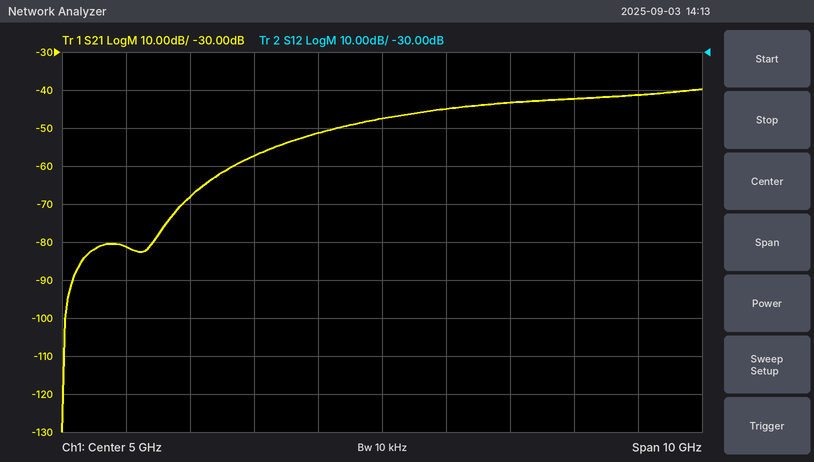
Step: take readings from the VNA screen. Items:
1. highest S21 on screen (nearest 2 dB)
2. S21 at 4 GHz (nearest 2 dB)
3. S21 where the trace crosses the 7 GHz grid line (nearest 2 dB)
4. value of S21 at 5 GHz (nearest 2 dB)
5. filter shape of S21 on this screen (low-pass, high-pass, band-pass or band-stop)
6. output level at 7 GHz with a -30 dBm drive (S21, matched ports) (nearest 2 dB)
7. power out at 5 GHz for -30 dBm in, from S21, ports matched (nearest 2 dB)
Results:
-40 dB
-52 dB
-44 dB
-48 dB
high-pass
-74 dBm
-78 dBm
